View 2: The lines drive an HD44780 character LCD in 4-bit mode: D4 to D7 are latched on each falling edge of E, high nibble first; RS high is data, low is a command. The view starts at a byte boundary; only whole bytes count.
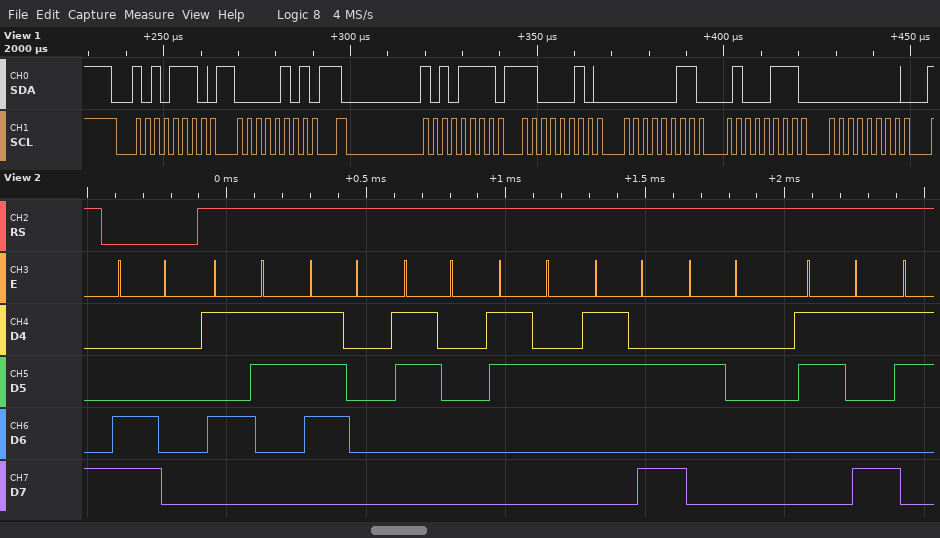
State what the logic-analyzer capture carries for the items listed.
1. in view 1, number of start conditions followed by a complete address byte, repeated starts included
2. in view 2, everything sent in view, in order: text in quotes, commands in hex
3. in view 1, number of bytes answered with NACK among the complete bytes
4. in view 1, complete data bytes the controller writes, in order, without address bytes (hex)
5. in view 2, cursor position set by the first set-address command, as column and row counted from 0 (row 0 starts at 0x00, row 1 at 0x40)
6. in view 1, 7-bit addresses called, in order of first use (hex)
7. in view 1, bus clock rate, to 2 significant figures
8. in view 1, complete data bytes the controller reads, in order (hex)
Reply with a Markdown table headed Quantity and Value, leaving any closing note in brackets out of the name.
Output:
| Quantity | Value |
|---|---|
| in view 1, number of start conditions followed by a complete address byte, repeated starts included | 2 |
| in view 2, everything sent in view, in order: text in quotes, commands in hex | 0xC0 "Sp02: 9" |
| in view 1, number of bytes answered with NACK among the complete bytes | 0 |
| in view 1, complete data bytes the controller writes, in order, without address bytes | 05 |
| in view 2, cursor position set by the first set-address command, as column and row counted from 0 | column 0, row 1 |
| in view 1, 7-bit addresses called, in order of first use | 0x57 |
| in view 1, bus clock rate, to 2 significant figures | 400 kHz |
| in view 1, complete data bytes the controller reads, in order | C2 03 47 00 |
